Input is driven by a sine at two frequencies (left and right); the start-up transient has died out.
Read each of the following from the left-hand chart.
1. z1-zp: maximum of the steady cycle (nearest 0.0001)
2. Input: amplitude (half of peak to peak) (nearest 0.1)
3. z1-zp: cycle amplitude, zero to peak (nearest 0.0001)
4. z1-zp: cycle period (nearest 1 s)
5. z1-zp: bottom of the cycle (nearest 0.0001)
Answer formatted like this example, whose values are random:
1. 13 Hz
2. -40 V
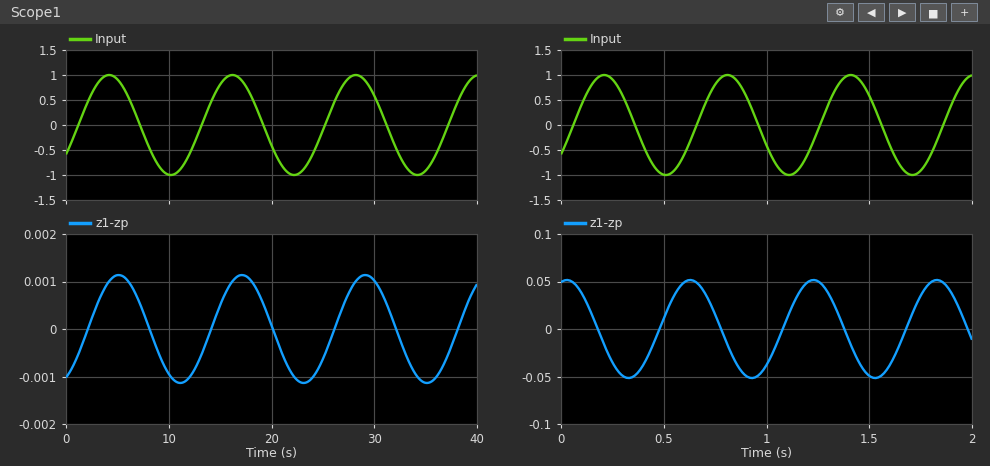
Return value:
1. 0.0011
2. 1.0
3. 0.0011
4. 12 s
5. -0.0011
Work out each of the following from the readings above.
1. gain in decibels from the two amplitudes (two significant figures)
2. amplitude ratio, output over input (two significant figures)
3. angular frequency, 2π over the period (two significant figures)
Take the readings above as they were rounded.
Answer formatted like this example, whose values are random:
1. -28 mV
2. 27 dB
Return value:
1. -59 dB
2. 0.0011
3. 0.52 rad/s
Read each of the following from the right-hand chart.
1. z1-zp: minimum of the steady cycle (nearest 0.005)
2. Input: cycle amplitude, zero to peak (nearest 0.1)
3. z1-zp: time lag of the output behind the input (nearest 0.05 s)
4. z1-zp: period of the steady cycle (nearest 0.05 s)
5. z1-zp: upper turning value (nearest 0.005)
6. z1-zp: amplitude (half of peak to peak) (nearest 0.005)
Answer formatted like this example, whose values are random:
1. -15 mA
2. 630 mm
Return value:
1. -0.050
2. 1.0
3. 0.40 s
4. 0.60 s
5. 0.050
6. 0.050
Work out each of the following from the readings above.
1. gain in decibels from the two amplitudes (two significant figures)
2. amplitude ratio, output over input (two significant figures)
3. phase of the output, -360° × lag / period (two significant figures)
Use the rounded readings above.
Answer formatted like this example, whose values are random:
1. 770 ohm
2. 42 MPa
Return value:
1. -26 dB
2. 0.050
3. -240°
